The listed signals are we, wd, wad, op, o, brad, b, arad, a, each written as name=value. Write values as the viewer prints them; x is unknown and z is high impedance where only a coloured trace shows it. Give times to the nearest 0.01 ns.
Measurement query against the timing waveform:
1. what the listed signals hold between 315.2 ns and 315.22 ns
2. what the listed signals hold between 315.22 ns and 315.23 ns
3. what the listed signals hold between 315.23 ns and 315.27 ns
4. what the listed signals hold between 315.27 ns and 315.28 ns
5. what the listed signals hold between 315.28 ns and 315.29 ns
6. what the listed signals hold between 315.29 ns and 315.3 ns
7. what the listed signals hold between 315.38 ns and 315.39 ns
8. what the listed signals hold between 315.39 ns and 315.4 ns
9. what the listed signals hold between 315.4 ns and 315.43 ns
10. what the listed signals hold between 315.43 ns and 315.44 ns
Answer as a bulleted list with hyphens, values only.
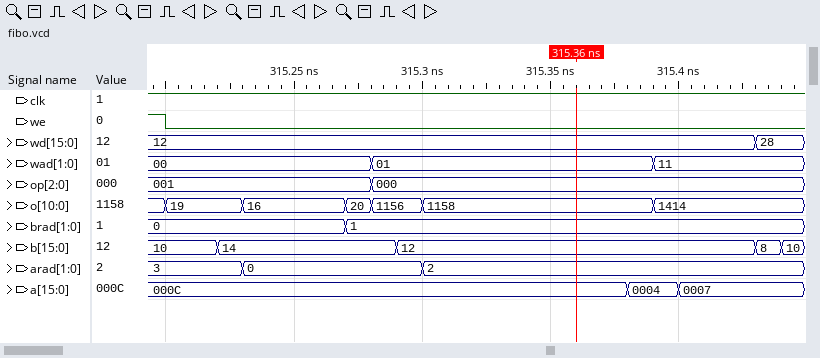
- we=0, wd=12, wad=00, op=001, o=19, brad=0, b=10, arad=3, a=000C
- we=0, wd=12, wad=00, op=001, o=19, brad=0, b=14, arad=3, a=000C
- we=0, wd=12, wad=00, op=001, o=16, brad=0, b=14, arad=0, a=000C
- we=0, wd=12, wad=00, op=001, o=20, brad=1, b=14, arad=0, a=000C
- we=0, wd=12, wad=01, op=000, o=1156, brad=1, b=14, arad=0, a=000C
- we=0, wd=12, wad=01, op=000, o=1156, brad=1, b=12, arad=0, a=000C
- we=0, wd=12, wad=01, op=000, o=1158, brad=1, b=12, arad=2, a=0004
- we=0, wd=12, wad=11, op=000, o=1414, brad=1, b=12, arad=2, a=0004
- we=0, wd=12, wad=11, op=000, o=1414, brad=1, b=12, arad=2, a=0007
- we=0, wd=28, wad=11, op=000, o=1414, brad=1, b=8, arad=2, a=0007
